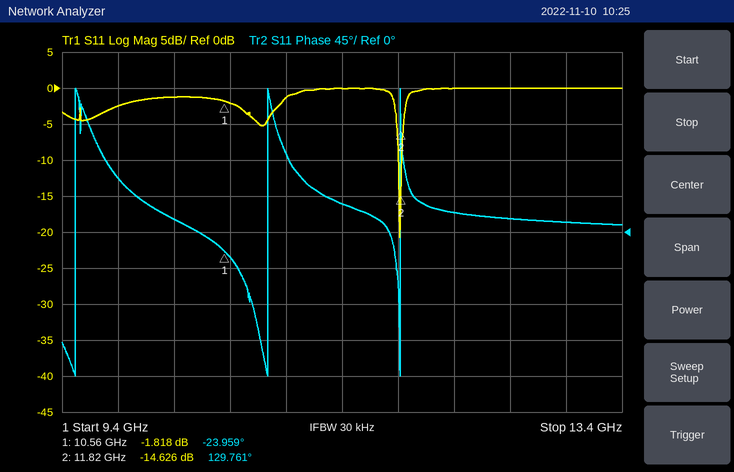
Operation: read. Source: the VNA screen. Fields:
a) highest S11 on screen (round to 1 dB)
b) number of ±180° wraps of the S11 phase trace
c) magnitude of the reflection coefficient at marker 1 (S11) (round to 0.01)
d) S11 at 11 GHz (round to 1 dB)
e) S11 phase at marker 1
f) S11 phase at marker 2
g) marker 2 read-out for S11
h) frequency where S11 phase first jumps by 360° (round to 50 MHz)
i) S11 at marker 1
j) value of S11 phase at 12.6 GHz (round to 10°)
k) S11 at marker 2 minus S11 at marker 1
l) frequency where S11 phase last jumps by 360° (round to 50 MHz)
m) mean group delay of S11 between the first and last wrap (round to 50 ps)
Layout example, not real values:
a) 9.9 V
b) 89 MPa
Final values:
a) 0 dB
b) 3
c) 0.81
d) -1 dB
e) -23.959°
f) 129.761°
g) -14.626 dB
h) 9.50 GHz
i) -1.818 dB
j) 20°
k) -12.808 dB
l) 11.80 GHz
m) 850 ps
